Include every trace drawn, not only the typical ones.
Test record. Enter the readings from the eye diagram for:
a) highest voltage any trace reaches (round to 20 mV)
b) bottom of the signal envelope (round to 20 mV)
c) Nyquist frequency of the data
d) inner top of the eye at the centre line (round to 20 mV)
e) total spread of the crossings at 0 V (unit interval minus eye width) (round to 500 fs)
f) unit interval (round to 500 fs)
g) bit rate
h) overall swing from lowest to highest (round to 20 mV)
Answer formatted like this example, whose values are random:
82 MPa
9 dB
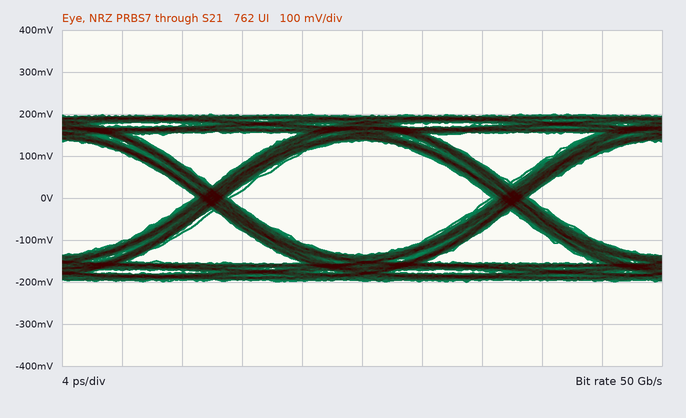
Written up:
200 mV
-200 mV
25 GHz
140 mV
2.5 ps
20.0 ps
50 Gb/s
400 mV
